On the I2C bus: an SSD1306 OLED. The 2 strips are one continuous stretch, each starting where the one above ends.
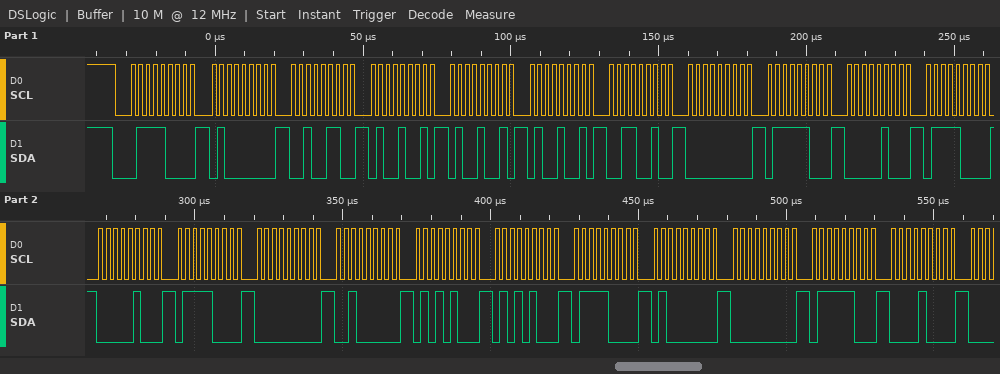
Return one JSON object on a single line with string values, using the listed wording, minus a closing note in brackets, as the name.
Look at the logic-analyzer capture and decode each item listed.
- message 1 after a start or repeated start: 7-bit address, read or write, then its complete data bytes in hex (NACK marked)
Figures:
{"message 1 after a start or repeated start: 7-bit address, read or write, then its complete data bytes in hex": "0x3C write: 40 26 49 49 49 32 00 7C 04 78 04 78 00 20 54 54 78 40 00 7C 08"}
